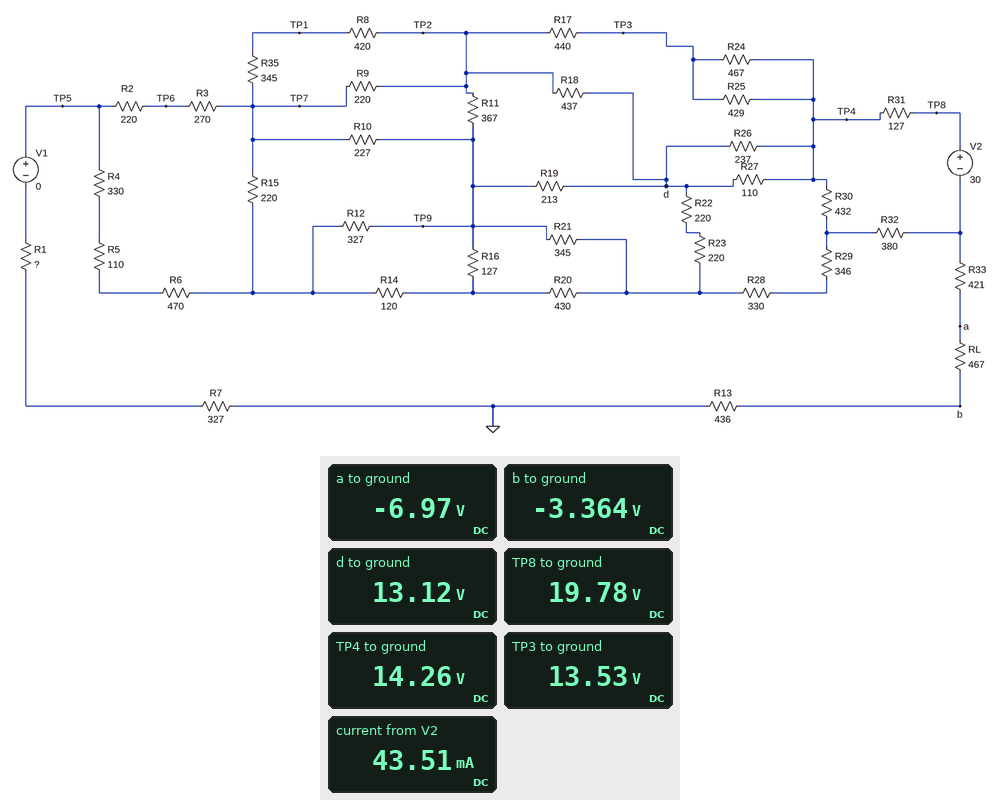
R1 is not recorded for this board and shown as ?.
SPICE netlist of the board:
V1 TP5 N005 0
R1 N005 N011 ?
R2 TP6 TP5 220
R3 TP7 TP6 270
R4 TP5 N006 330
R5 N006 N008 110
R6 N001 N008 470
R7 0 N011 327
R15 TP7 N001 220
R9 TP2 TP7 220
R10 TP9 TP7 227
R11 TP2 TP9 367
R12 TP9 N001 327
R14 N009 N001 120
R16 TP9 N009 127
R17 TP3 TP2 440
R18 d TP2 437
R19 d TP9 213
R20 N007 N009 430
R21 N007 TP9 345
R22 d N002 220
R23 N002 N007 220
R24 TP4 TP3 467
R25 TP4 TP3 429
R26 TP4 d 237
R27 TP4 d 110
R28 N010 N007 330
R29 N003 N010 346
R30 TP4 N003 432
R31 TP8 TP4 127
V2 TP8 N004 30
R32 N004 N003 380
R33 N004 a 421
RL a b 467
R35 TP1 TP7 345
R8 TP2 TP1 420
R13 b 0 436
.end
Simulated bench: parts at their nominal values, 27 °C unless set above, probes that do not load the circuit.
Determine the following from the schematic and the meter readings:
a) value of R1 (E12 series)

820 Ω
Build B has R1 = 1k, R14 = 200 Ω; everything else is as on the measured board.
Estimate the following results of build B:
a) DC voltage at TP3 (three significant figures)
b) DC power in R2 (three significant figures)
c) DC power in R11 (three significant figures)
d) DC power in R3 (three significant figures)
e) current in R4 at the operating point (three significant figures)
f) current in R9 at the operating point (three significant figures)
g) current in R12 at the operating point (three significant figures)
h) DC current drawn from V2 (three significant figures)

14.2 V
5.14 mW
547 µW
6.31 mW
2.45 mA
3.29 mA
1.27 mA
43.2 mA
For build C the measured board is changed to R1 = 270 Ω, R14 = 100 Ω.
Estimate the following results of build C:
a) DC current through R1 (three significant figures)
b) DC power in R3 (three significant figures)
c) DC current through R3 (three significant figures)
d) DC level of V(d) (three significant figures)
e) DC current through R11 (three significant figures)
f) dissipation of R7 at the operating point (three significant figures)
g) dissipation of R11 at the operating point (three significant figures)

9.40 mA
10.3 mW
6.18 mA
10.6 V
1.26 mA
28.9 mW
585 µW
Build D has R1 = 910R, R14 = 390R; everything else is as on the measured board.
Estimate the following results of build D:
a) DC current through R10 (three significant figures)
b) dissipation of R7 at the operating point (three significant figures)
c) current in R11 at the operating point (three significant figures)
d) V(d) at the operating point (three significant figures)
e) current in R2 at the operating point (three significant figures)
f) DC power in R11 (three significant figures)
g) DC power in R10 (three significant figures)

1.32 mA
18.3 mW
1.21 mA
13.5 V
4.98 mA
534 µW
397 µW
